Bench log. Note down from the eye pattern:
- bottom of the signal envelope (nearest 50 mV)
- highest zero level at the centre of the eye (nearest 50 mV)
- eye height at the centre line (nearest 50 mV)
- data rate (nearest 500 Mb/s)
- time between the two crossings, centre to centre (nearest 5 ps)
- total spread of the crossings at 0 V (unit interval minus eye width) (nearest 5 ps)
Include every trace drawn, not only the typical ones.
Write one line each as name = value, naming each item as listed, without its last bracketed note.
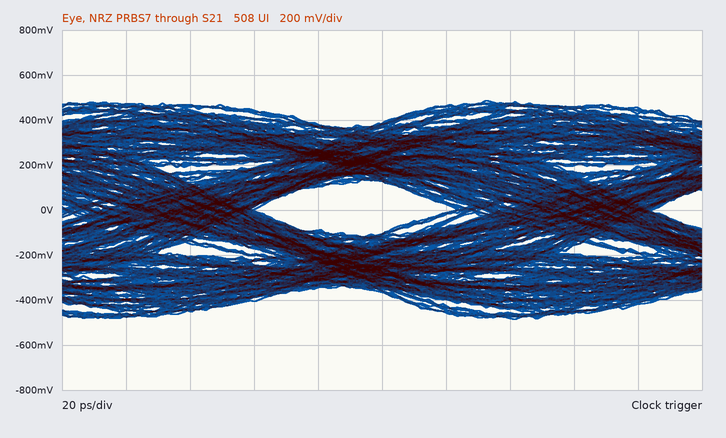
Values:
bottom of the signal envelope = -500 mV
highest zero level at the centre of the eye = -100 mV
eye height at the centre line = 250 mV
data rate = 8.0 Gb/s
time between the two crossings, centre to centre = 125 ps
total spread of the crossings at 0 V (unit interval minus eye width) = 60 ps
